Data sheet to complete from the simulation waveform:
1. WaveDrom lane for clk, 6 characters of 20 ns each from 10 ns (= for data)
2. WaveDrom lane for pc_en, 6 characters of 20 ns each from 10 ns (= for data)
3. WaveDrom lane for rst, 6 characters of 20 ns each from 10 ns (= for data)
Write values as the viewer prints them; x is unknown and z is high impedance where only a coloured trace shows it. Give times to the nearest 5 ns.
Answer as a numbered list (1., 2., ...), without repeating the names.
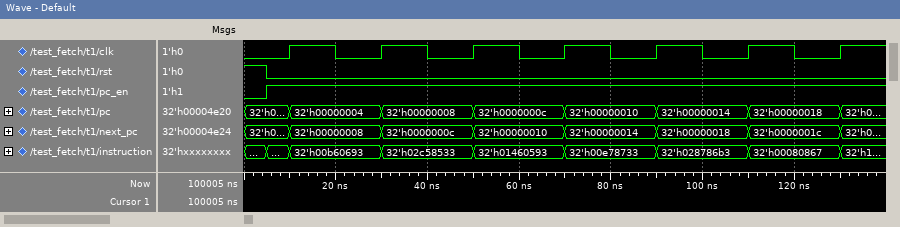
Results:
1. {name: 'clk', wave: 'p.....'}
2. {name: 'pc_en', wave: '1.....'}
3. {name: 'rst', wave: '0.....'}
